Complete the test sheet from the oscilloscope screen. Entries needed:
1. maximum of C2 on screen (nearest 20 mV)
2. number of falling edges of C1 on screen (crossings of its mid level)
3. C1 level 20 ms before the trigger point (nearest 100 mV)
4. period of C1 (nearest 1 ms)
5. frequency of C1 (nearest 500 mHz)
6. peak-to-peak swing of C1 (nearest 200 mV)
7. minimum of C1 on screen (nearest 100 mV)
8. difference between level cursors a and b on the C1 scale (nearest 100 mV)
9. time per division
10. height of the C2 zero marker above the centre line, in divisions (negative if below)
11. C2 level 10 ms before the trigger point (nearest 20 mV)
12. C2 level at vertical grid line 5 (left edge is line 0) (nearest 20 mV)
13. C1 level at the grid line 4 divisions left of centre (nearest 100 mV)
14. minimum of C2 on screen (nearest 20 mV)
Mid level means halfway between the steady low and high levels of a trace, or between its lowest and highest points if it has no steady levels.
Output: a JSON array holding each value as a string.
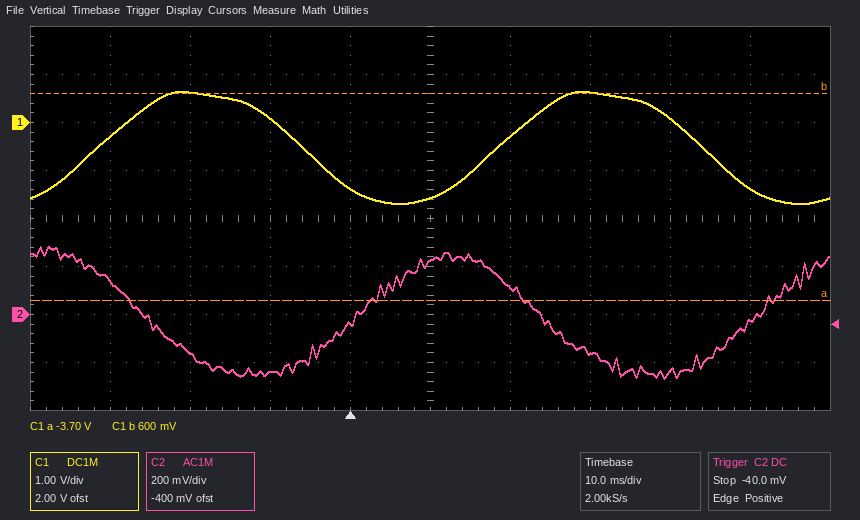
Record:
["280 mV", "2", "600 mV", "50 ms", "20.0 Hz", "2.4 V", "-1.7 V", "4.3 V", "10 ms", "-2.0 div", "-240 mV", "220 mV", "-300 mV", "-260 mV"]
